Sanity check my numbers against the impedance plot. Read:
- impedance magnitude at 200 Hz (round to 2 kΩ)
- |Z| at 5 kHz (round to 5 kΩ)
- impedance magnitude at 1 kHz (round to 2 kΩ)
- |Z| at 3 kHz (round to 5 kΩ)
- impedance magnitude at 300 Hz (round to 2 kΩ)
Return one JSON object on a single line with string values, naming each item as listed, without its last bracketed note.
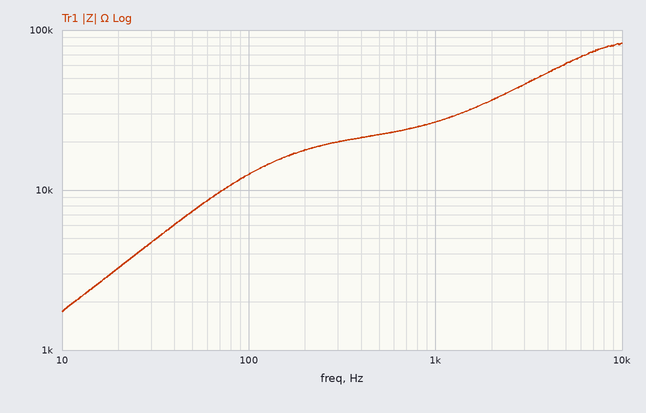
{"impedance magnitude at 200 Hz": "18 kΩ", "|Z| at 5 kHz": "60 kΩ", "impedance magnitude at 1 kHz": "26 kΩ", "|Z| at 3 kHz": "45 kΩ", "impedance magnitude at 300 Hz": "20 kΩ"}
